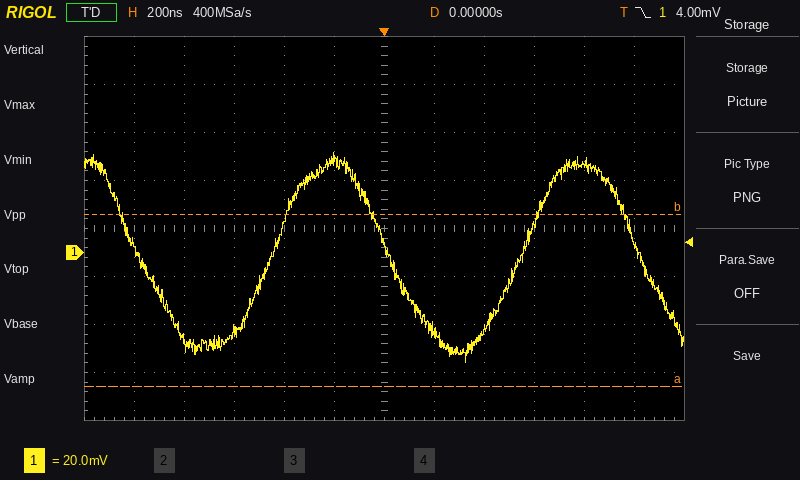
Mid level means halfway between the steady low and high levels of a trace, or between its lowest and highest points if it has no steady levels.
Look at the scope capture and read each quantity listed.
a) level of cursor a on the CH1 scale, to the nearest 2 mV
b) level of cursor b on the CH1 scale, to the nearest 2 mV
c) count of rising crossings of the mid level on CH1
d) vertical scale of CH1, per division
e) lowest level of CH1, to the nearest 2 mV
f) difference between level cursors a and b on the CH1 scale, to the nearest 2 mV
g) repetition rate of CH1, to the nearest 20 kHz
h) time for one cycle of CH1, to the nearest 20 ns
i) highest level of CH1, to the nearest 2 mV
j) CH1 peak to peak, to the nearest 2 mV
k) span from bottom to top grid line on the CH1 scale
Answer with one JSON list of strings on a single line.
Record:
["-56 mV", "16 mV", "2", "20 mV", "-46 mV", "72 mV", "1.00 MHz", "1.00 µs", "42 mV", "88 mV", "160 mV"]
